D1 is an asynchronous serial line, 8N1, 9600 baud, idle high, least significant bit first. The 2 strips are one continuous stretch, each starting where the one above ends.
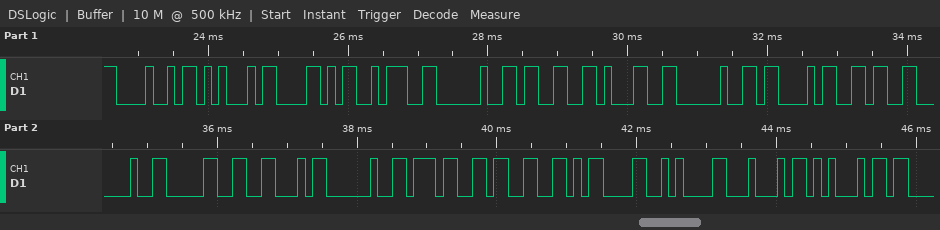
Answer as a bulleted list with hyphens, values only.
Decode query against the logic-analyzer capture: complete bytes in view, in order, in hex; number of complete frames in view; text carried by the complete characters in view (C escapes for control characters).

- 0x48 0x45 0x58 0x3A 0x20 0x33 0x31 0x20 0x43 0x36 0x20 0x30 0x46 0x20 0x37 0x33 0x0D 0x0A 0x44 0x45
- 20
- "HEX: 31 C6 0F 73\r\nDE"
